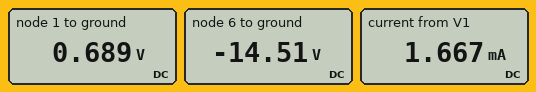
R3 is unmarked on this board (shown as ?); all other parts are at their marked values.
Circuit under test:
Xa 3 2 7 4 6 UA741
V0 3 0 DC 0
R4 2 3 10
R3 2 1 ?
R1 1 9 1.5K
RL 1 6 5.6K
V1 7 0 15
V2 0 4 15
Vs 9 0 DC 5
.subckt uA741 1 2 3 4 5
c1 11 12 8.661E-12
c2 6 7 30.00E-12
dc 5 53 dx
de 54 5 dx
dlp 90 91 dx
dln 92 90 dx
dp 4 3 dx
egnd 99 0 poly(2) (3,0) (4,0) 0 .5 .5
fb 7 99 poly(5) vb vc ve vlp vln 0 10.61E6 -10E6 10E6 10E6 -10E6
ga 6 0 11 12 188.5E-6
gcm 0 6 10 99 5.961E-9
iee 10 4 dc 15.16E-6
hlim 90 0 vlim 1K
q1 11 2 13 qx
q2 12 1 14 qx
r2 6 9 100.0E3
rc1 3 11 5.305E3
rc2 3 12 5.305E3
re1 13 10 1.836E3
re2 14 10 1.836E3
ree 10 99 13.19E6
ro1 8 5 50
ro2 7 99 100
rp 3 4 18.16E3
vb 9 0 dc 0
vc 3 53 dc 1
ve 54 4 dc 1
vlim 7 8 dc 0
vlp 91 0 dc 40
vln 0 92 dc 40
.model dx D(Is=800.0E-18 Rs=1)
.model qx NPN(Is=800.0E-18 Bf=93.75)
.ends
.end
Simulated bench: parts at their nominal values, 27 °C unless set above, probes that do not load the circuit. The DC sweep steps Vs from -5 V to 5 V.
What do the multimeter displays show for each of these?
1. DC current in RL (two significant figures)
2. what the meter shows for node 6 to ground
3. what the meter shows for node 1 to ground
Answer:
2.7 mA
-14.51 V
0.689 V
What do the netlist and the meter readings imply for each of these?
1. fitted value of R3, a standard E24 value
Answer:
4.3 kΩ
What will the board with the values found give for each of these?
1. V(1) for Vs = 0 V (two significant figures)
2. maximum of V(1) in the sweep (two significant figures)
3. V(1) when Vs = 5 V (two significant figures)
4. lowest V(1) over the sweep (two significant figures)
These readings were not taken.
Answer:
8.5 mV
690 mV
690 mV
-690 mV
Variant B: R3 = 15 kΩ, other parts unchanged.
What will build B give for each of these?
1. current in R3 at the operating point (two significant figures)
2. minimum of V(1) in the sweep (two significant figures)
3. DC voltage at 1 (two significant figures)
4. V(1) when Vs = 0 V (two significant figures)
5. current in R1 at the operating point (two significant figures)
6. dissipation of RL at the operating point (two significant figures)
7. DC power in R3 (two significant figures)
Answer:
55 µA
-820 mV
820 mV
29 mV
2.8 mA
42 mW
45 µW
